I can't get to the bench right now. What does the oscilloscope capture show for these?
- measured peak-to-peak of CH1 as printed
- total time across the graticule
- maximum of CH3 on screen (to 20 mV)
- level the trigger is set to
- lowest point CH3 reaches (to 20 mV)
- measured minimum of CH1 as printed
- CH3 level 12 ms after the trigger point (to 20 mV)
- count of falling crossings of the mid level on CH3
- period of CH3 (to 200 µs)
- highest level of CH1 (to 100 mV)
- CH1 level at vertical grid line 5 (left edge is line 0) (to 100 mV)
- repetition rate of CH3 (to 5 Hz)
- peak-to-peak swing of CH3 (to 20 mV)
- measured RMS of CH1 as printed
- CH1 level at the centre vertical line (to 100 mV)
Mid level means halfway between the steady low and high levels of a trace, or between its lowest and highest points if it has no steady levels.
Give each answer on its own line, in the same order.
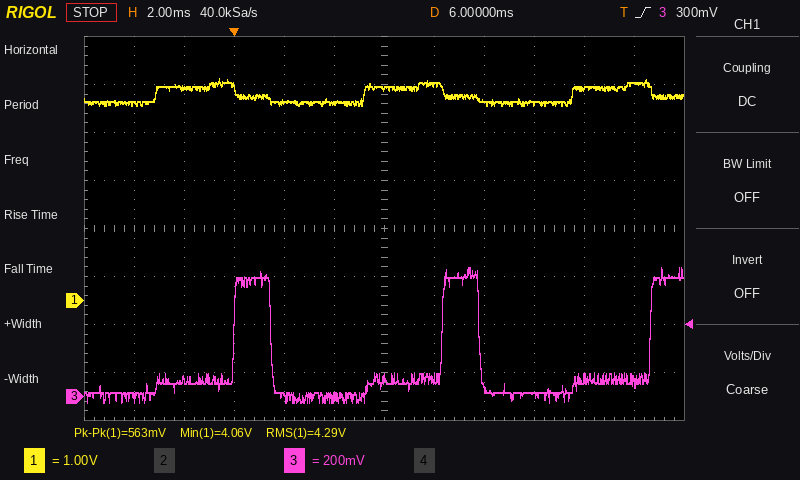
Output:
563 mV
24 ms
540 mV
300 mV
-20 mV
4.06 V
0 mV
2
8.4 ms
4.6 V
4.1 V
120 Hz
560 mV
4.29 V
4.4 V
